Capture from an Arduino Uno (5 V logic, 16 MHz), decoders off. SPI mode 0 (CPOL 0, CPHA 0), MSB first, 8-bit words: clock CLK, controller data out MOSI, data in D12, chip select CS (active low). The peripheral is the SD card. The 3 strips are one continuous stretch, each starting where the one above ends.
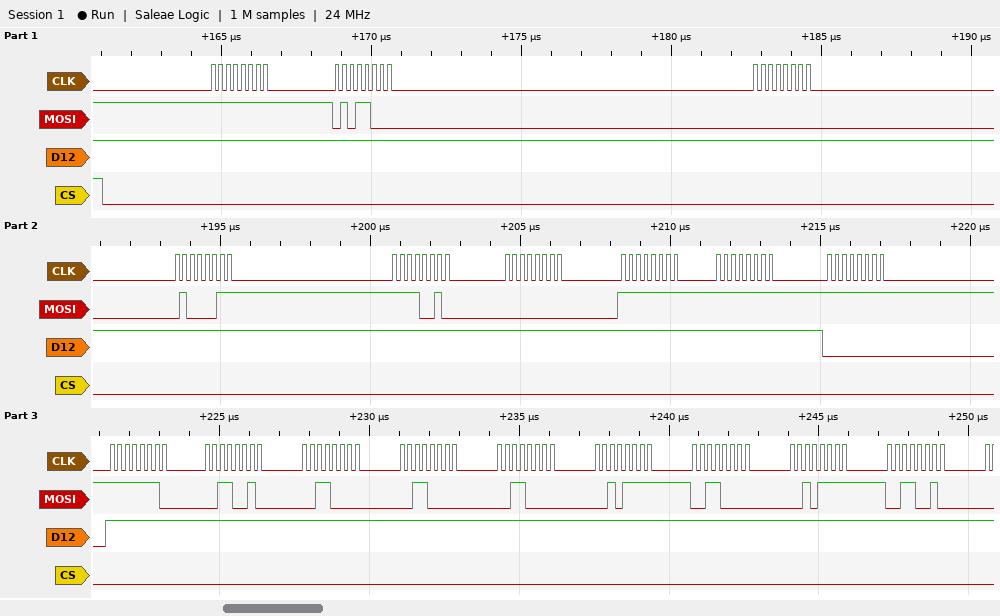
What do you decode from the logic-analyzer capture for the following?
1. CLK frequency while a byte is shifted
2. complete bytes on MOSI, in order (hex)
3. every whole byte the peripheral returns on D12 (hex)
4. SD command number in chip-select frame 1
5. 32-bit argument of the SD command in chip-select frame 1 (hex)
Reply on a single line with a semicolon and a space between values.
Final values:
4 MHz; 0xFF 0x58 0x00 0x43 0xF2 0x00 0xFF 0xFF 0xFF 0xFE 0x32 0x30 0x30 0x30 0x2F 0x30 0x2F 0x32; 0xFF 0xFF 0xFF 0xFF 0xFF 0xFF 0xFF 0xFF 0x00 0xFF 0xFF 0xFF 0xFF 0xFF 0xFF 0xFF 0xFF 0xFF; CMD24; 0x0043F200
